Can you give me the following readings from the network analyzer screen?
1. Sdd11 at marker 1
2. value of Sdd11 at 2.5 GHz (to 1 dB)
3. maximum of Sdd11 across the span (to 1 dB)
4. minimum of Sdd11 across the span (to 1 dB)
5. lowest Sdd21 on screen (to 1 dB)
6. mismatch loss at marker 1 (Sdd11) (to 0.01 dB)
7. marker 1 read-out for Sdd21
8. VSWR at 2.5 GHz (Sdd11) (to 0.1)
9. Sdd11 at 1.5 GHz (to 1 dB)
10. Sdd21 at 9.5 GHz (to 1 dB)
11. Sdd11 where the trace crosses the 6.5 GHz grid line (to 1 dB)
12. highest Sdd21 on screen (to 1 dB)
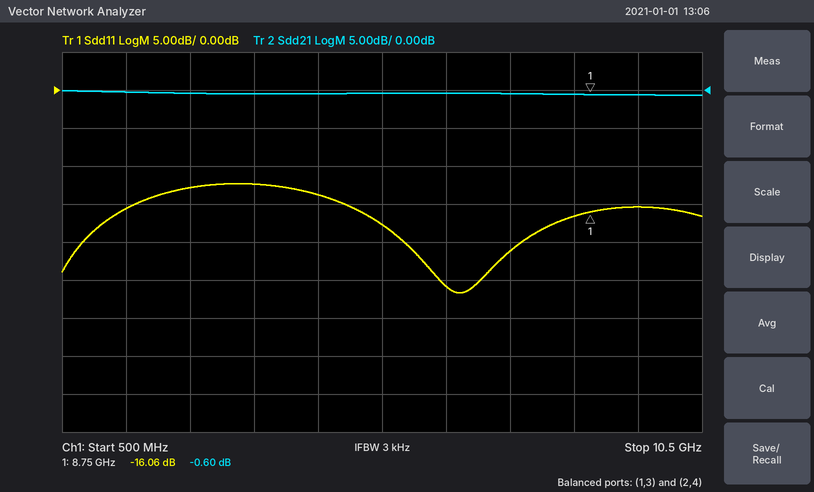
-16.06 dB
-13 dB
-12 dB
-27 dB
-1 dB
0.11 dB
-0.60 dB
1.6
-16 dB
-1 dB
-26 dB
0 dB
